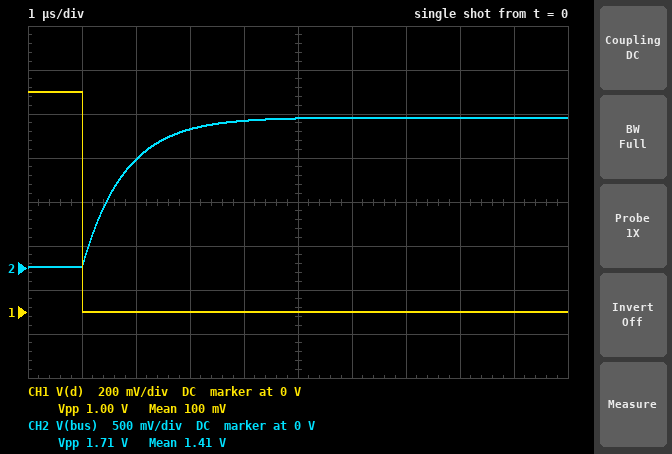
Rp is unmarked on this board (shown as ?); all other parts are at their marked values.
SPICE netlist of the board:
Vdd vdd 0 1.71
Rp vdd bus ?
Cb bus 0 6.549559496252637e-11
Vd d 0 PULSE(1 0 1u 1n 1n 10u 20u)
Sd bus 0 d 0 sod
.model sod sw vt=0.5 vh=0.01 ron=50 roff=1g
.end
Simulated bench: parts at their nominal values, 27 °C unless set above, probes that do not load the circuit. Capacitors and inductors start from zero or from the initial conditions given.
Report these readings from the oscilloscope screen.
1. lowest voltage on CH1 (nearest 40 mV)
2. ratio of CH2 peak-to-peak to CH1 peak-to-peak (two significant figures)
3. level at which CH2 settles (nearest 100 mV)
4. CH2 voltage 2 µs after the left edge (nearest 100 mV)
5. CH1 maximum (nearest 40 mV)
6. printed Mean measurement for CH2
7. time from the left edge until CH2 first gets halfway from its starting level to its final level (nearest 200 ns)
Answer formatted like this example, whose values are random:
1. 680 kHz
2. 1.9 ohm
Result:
1. 0 V
2. 1.7
3. 1.7 V
4. 1.2 V
5. 1.00 V
6. 1.41 V
7. 1.6 µs
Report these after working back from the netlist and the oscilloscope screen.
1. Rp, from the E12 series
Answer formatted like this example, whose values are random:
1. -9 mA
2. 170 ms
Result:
1. 12 kΩ
